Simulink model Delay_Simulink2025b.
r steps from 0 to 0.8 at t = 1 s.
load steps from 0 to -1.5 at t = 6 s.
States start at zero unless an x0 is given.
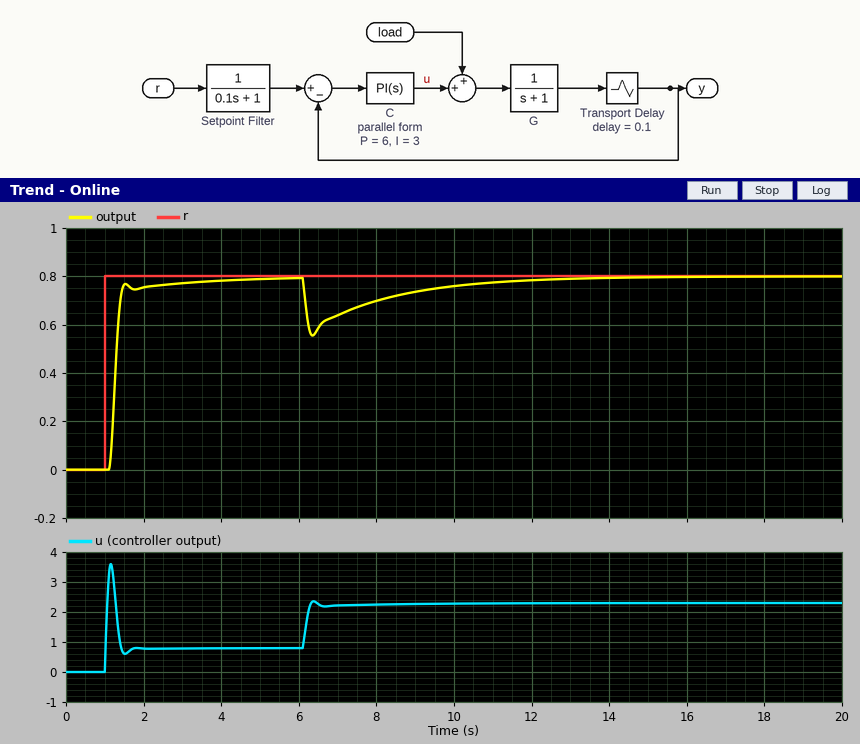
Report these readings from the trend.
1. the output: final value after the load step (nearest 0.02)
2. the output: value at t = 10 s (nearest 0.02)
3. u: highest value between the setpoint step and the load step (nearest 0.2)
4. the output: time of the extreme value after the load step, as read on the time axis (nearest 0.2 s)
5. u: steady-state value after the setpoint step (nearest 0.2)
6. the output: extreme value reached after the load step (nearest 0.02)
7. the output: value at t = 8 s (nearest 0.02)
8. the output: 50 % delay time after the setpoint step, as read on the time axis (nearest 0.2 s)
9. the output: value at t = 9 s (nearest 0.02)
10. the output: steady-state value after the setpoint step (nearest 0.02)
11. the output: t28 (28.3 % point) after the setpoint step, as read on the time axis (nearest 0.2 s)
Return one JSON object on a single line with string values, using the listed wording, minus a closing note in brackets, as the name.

{"the output: final value after the load step": "0.80", "the output: value at t = 10 s": "0.76", "u: highest value between the setpoint step and the load step": "3.6", "the output: time of the extreme value after the load step, as read on the time axis": "6.4 s", "u: steady-state value after the setpoint step": "0.8", "the output: extreme value reached after the load step": "0.56", "the output: value at t = 8 s": "0.70", "the output: 50 % delay time after the setpoint step, as read on the time axis": "1.2 s", "the output: value at t = 9 s": "0.74", "the output: steady-state value after the setpoint step": "0.80", "the output: t28 (28.3 % point) after the setpoint step, as read on the time axis": "1.2 s"}
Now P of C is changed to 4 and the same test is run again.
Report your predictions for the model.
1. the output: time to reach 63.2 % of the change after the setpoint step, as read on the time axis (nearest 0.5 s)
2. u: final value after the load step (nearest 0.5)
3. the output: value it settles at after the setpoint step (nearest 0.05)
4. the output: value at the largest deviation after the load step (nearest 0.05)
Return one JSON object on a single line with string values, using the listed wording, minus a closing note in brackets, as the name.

{"the output: time to reach 63.2 % of the change after the setpoint step, as read on the time axis": "1.5 s", "u: final value after the load step": "2.5", "the output: value it settles at after the setpoint step": "0.80", "the output: value at the largest deviation after the load step": "0.50"}
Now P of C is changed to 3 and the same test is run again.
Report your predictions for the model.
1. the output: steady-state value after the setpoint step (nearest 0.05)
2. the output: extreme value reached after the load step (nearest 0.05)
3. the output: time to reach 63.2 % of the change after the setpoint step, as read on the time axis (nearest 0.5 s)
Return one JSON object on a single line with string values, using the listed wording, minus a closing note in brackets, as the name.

{"the output: steady-state value after the setpoint step": "0.80", "the output: extreme value reached after the load step": "0.45", "the output: time to reach 63.2 % of the change after the setpoint step, as read on the time axis": "1.5 s"}
